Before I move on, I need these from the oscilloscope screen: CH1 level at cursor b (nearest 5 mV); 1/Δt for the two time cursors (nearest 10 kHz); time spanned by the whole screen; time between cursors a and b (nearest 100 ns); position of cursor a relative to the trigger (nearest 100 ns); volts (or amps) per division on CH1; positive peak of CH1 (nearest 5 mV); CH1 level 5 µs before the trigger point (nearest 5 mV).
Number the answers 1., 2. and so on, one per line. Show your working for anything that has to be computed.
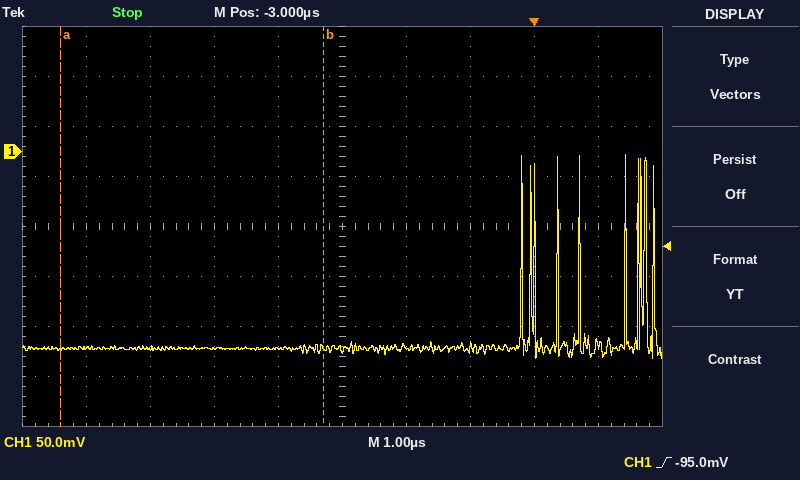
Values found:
1. -195 mV
2. 1 / 4.1 µs ≈ 240 kHz
3. 10 µs
4. 4.1 µs
5. -7.4 µs
6. 50 mV
7. -5 mV
8. -195 mV
